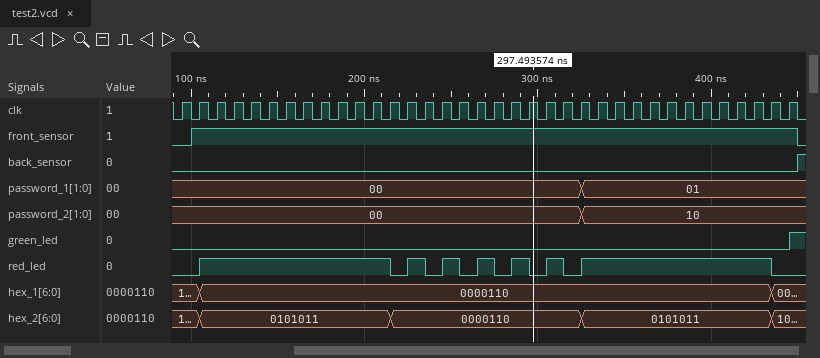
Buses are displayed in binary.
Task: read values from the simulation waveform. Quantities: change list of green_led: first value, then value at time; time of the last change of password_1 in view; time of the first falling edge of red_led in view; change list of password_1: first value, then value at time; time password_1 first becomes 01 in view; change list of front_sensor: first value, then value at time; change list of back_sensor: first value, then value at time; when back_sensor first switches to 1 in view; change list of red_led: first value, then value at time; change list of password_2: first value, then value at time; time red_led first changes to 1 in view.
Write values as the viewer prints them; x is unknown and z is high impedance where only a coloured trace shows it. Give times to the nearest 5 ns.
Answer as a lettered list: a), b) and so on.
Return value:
a) 0, 1 at 445 ns
b) 325 ns
c) 215 ns
d) 00, 01 at 325 ns
e) 325 ns
f) 0, 1 at 100 ns, 0 at 450 ns
g) 0, 1 at 450 ns
h) 450 ns
i) 0, 1 at 105 ns, 0 at 215 ns, 1 at 225 ns, 0 at 235 ns, 1 at 245 ns, 0 at 255 ns, 1 at 265 ns, 0 at 275 ns, 1 at 285 ns, 0 at 295 ns, 1 at 305 ns, 0 at 315 ns, 1 at 325 ns, 0 at 435 ns
j) 00, 10 at 325 ns
k) 105 ns
